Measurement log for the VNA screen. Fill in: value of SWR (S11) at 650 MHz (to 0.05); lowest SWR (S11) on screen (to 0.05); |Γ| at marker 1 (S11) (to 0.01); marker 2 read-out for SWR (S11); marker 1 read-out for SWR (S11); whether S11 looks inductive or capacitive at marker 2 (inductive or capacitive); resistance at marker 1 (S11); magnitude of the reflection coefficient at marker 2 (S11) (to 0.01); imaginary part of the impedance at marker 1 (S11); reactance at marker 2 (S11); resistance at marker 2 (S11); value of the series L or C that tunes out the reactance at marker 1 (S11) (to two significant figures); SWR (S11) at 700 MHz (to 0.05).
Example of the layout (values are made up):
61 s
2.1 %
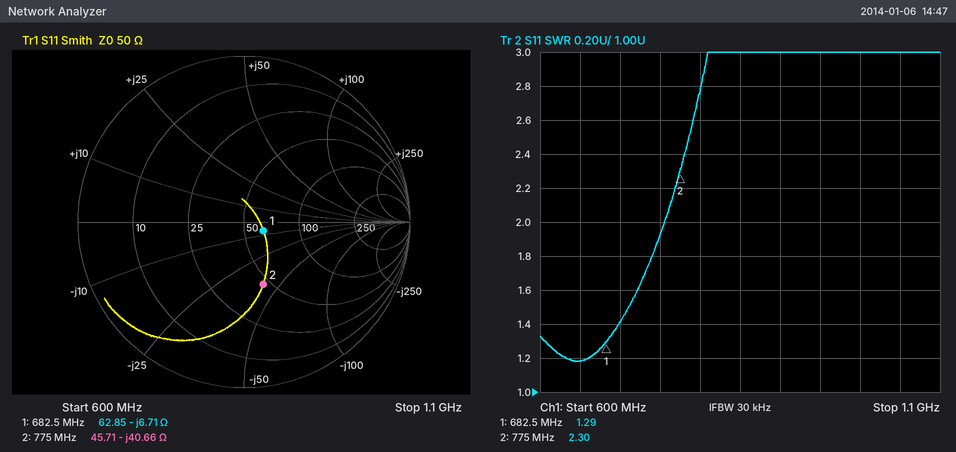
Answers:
1.20
1.20
0.13
2.30
1.29
capacitive
62.85 Ω
0.39
-6.71 Ω
-40.66 Ω
45.71 Ω
1.6 nH
1.40
